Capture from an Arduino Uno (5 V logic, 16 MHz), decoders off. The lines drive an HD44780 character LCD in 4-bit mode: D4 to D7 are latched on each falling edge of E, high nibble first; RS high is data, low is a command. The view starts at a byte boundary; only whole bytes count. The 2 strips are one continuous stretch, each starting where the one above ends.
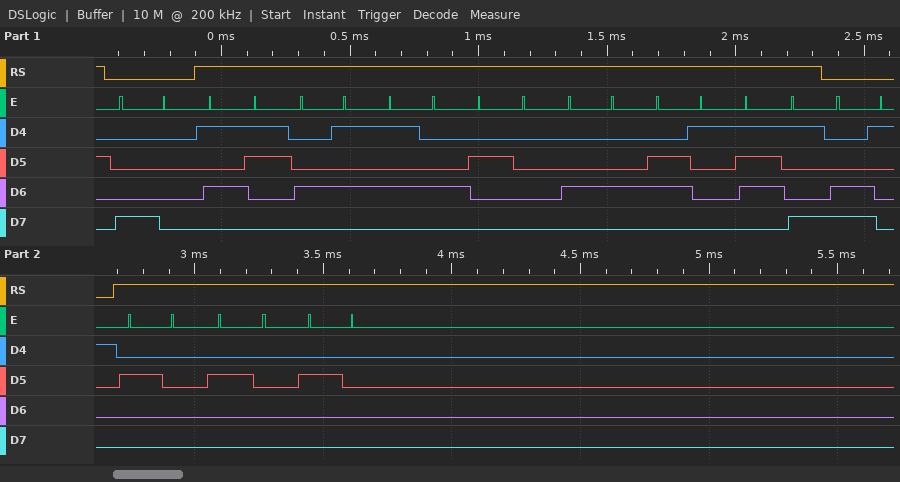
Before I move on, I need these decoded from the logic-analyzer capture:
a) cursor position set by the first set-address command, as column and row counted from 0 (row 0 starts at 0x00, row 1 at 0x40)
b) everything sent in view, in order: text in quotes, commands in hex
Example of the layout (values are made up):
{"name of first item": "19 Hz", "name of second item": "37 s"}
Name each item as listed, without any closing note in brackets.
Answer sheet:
{"cursor position set by the first set-address command, as column and row counted from 0": "column 0, row 0", "everything sent in view, in order: text in quotes, commands in hex": "0x80 \"SET Day\" 0xC1 \"   \""}
